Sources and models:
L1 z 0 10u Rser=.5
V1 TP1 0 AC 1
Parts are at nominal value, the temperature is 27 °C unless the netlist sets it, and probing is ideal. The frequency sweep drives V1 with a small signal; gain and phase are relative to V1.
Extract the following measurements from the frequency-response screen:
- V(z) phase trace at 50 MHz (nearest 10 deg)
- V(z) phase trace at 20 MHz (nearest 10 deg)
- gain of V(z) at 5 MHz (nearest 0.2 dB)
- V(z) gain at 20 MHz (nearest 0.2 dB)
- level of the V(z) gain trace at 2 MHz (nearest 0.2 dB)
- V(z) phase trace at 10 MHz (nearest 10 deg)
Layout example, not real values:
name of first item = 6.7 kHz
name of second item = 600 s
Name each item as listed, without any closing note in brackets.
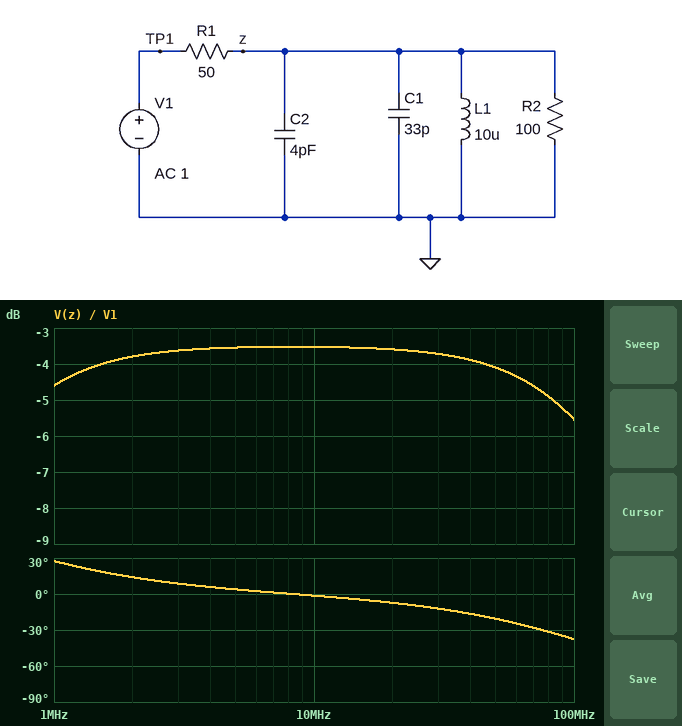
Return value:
V(z) phase trace at 50 MHz = -20 deg
V(z) phase trace at 20 MHz = -10 deg
gain of V(z) at 5 MHz = -3.6 dB
V(z) gain at 20 MHz = -3.6 dB
level of the V(z) gain trace at 2 MHz = -3.8 dB
V(z) phase trace at 10 MHz = 0 deg
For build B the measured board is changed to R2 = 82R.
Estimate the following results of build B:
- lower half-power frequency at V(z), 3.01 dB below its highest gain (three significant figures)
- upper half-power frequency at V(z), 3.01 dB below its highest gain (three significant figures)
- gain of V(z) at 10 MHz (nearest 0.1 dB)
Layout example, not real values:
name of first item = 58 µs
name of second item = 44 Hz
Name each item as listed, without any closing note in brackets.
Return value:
lower half-power frequency at V(z), 3.01 dB below its highest gain = 500 kHz
upper half-power frequency at V(z), 3.01 dB below its highest gain = 139 MHz
gain of V(z) at 10 MHz = -4.1 dB
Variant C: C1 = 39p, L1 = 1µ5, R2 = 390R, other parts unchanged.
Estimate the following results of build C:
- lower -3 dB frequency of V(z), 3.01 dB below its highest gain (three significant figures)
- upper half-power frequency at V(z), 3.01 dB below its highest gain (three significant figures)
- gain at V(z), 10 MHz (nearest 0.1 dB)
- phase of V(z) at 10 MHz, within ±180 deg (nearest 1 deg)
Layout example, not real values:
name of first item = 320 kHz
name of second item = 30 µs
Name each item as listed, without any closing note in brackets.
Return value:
lower -3 dB frequency of V(z), 3.01 dB below its highest gain = 4.51 MHz
upper half-power frequency at V(z), 3.01 dB below its highest gain = 88.1 MHz
gain at V(z), 10 MHz = -1.6 dB
phase of V(z) at 10 MHz, within ±180 deg = 19 deg
